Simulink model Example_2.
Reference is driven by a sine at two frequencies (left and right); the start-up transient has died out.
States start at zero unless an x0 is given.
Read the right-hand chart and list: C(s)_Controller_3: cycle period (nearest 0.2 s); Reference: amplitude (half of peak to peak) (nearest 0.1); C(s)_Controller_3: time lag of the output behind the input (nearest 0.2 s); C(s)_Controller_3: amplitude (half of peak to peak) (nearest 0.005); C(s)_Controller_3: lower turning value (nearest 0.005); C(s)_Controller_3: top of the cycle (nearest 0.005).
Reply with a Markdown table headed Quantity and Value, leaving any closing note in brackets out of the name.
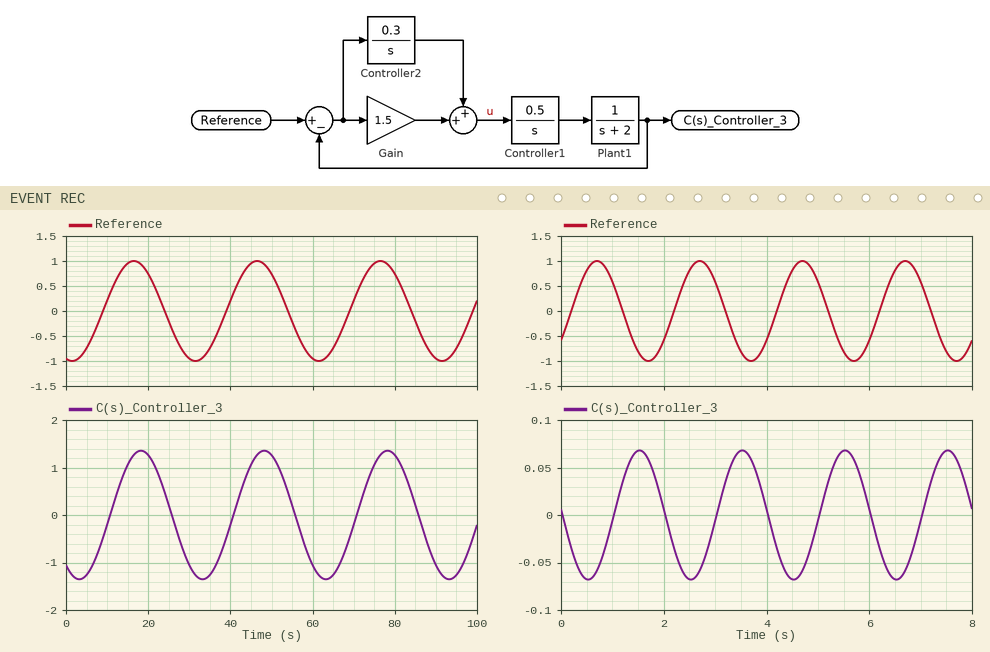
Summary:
| Quantity | Value |
|---|---|
| C(s)_Controller_3: cycle period | 2.0 s |
| Reference: amplitude (half of peak to peak) | 1.0 |
| C(s)_Controller_3: time lag of the output behind the input | 0.8 s |
| C(s)_Controller_3: amplitude (half of peak to peak) | 0.070 |
| C(s)_Controller_3: lower turning value | -0.070 |
| C(s)_Controller_3: top of the cycle | 0.070 |
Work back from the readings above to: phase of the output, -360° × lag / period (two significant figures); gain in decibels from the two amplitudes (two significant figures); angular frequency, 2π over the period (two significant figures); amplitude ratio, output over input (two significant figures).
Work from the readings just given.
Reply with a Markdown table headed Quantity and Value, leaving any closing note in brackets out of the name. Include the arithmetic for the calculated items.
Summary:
| Quantity | Value |
|---|---|
| phase of the output, -360° × lag / period | -360 × 0.8 / 2 = -140° |
| gain in decibels from the two amplitudes | 20 log10(0.07 / 1) = -23 dB |
| angular frequency, 2π over the period | 2π / 2 = 3.1 rad/s |
| amplitude ratio, output over input | 0.07 / 1 = 0.070 |
